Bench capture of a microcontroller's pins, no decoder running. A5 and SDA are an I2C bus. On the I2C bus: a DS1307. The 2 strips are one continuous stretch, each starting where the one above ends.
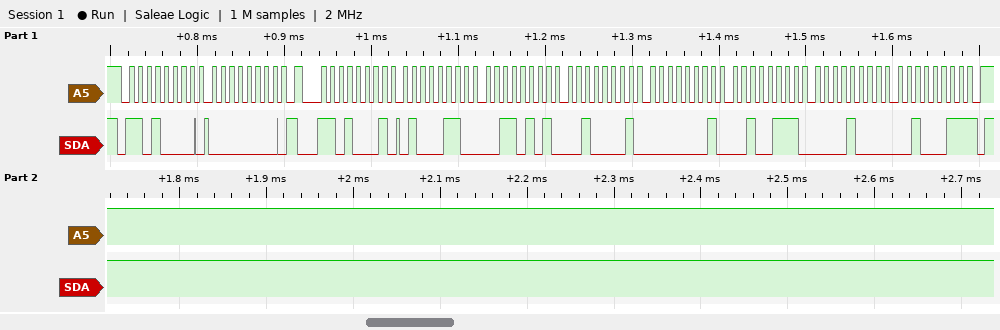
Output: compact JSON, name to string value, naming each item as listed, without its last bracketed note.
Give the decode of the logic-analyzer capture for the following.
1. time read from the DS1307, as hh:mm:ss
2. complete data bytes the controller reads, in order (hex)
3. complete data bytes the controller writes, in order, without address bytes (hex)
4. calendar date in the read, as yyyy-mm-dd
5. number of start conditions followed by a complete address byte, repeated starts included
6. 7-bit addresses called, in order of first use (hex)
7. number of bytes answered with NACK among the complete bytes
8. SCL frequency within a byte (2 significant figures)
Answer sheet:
{"time read from the DS1307, as hh:mm:ss": "21:35:46", "complete data bytes the controller reads, in order": "46 35 21 01 27 08 23", "complete data bytes the controller writes, in order, without address bytes": "00", "calendar date in the read, as yyyy-mm-dd": "2023-08-27", "number of start conditions followed by a complete address byte, repeated starts included": "2", "7-bit addresses called, in order of first use": "0x68", "number of bytes answered with NACK among the complete bytes": "1", "SCL frequency within a byte": "100 kHz"}
